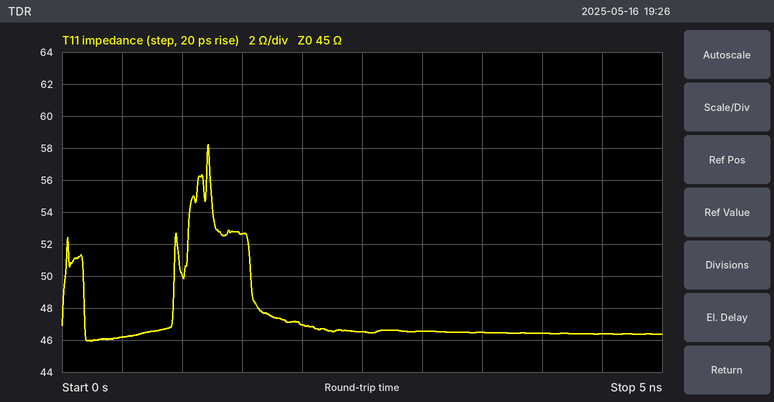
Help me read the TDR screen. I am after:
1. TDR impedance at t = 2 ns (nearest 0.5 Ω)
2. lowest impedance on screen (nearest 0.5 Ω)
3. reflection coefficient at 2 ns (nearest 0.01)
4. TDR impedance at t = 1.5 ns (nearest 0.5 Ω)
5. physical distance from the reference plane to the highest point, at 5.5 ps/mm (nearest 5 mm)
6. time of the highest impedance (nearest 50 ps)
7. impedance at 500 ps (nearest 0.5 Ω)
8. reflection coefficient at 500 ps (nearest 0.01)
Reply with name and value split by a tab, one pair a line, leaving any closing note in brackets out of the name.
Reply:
TDR impedance at t = 2 ns	47.0 Ω
lowest impedance on screen	46.0 Ω
reflection coefficient at 2 ns	+0.02
TDR impedance at t = 1.5 ns	52.5 Ω
physical distance from the reference plane to the highest point, at 5.5 ps/mm	110 mm
time of the highest impedance	1.20 ns
impedance at 500 ps	46.0 Ω
reflection coefficient at 500 ps	+0.01
